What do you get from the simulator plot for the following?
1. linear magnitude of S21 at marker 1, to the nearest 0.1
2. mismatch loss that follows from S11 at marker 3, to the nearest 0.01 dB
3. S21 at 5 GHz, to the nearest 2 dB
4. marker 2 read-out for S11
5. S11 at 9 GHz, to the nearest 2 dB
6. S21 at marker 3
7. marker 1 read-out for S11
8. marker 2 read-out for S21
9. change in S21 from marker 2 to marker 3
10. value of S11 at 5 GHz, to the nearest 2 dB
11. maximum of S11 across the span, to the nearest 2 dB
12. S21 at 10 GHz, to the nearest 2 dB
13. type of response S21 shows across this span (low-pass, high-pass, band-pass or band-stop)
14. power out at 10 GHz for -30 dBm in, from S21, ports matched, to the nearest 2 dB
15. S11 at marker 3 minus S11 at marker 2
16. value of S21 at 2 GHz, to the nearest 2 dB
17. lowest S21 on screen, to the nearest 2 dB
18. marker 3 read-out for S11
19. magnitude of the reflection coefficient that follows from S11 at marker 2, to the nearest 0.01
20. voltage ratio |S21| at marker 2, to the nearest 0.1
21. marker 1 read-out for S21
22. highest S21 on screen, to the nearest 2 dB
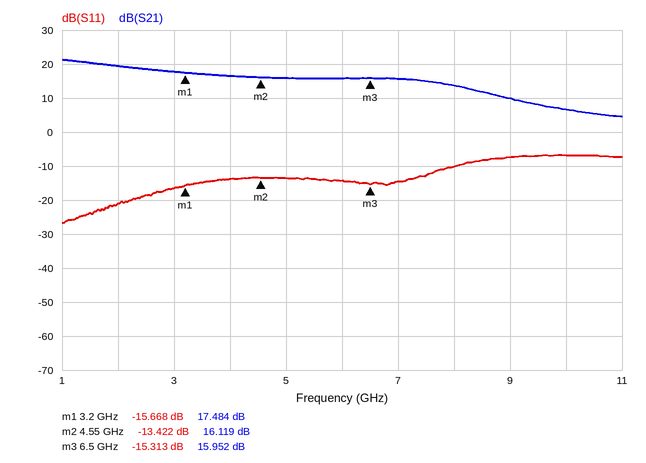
7.5
0.13 dB
16 dB
-13.422 dB
-8 dB
15.952 dB
-15.668 dB
16.119 dB
-0.167 dB
-14 dB
-6 dB
6 dB
low-pass
-24 dBm
-1.891 dB
20 dB
4 dB
-15.313 dB
0.21
6.4
17.484 dB
22 dB
